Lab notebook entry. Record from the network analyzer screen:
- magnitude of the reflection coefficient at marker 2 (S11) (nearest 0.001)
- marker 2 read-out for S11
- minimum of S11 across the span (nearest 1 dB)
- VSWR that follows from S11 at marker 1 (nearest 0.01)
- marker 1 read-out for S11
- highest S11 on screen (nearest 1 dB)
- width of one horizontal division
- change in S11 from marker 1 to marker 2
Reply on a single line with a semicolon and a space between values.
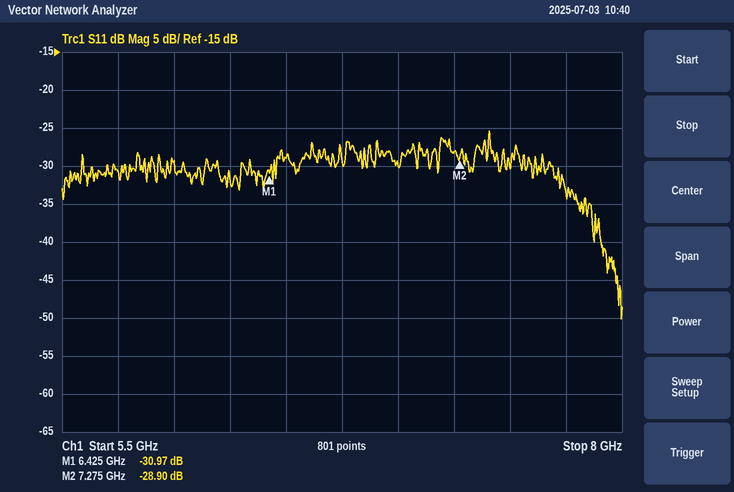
0.036; -28.90 dB; -50 dB; 1.06; -30.97 dB; -25 dB; 250 MHz; 2.07 dB
